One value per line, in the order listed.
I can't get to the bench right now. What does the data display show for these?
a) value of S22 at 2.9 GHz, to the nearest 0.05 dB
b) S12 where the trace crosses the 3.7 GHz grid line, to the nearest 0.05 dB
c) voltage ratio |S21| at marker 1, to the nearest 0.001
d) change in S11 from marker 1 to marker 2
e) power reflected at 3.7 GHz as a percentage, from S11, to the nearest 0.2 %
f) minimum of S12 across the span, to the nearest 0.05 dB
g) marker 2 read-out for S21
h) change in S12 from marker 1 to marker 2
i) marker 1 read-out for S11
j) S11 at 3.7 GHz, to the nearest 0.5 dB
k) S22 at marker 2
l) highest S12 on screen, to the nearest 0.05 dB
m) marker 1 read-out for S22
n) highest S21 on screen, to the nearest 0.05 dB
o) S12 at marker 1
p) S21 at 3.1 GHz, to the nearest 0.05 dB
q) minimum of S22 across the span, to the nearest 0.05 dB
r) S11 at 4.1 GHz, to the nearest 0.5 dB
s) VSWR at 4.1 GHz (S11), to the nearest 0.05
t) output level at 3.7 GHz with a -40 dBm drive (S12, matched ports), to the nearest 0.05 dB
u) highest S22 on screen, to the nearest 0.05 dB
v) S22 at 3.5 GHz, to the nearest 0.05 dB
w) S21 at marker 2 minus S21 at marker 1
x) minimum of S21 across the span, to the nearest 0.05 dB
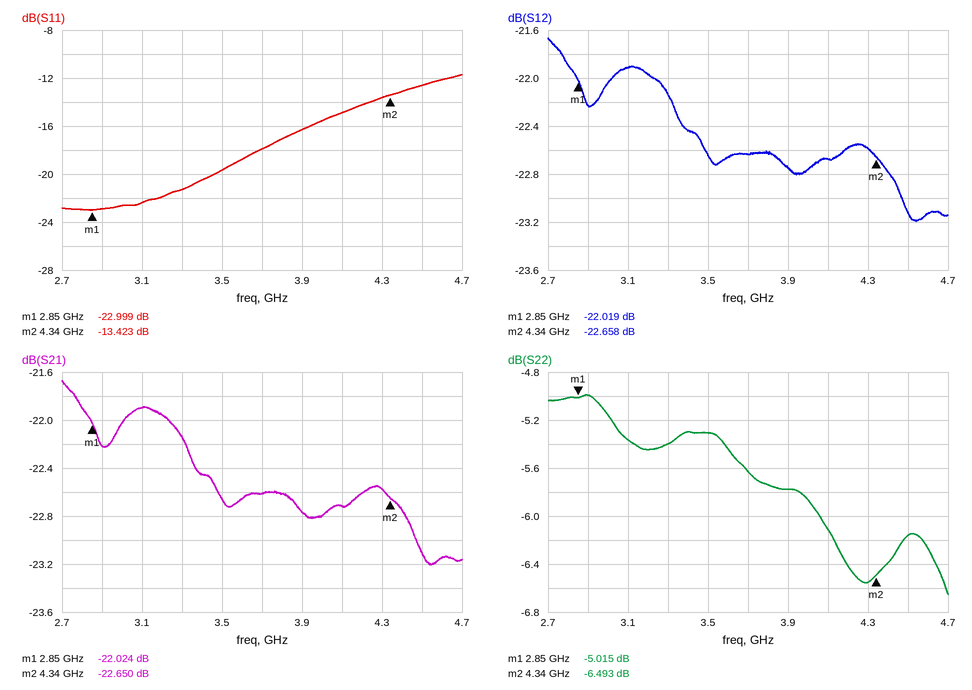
-5.00 dB
-22.65 dB
0.079
9.576 dB
1.6 %
-23.20 dB
-22.650 dB
-0.639 dB
-22.999 dB
-18.0 dB
-6.493 dB
-21.65 dB
-5.015 dB
-21.65 dB
-22.019 dB
-21.90 dB
-6.65 dB
-15.0 dB
1.45
-62.65 dBm
-5.00 dB
-5.30 dB
-0.626 dB
-23.20 dB
